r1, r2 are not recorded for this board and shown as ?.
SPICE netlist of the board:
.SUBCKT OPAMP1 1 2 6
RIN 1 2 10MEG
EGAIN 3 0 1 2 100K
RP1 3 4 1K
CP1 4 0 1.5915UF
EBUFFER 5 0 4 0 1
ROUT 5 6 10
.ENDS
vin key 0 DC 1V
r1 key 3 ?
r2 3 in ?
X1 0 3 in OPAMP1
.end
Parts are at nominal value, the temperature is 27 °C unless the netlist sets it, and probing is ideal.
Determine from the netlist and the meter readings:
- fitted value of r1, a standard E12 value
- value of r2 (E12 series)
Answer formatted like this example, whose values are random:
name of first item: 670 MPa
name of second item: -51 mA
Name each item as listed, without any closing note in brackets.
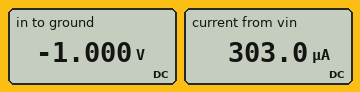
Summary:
fitted value of r1, a standard E12 value: 3.3 kΩ
value of r2: 3.3 kΩ
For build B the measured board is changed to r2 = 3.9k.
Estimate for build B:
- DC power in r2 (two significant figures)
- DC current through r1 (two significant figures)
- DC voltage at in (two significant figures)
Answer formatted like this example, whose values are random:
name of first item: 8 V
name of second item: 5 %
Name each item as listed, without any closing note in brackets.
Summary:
DC power in r2: 360 µW
DC current through r1: 300 µA
DC voltage at in: -1.2 V
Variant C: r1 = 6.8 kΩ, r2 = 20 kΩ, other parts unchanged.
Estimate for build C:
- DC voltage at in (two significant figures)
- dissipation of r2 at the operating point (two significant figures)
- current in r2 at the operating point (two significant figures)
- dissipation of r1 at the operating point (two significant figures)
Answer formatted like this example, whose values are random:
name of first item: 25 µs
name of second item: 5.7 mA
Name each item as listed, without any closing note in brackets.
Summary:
DC voltage at in: -2.9 V
dissipation of r2 at the operating point: 430 µW
current in r2 at the operating point: 150 µA
dissipation of r1 at the operating point: 150 µW
